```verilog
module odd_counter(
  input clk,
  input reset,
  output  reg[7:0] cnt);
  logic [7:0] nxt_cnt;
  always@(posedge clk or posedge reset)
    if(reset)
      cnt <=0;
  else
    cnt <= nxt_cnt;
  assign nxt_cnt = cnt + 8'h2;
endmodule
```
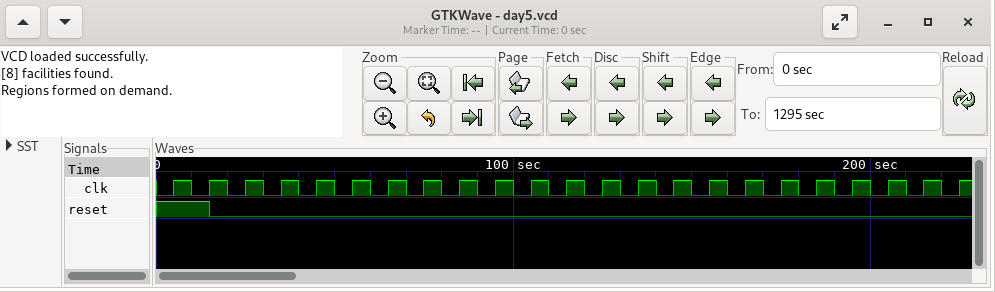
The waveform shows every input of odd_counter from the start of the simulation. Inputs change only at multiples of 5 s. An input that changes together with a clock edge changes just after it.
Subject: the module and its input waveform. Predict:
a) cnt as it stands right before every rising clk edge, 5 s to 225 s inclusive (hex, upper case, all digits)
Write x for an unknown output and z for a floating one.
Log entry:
00, 00, 00, 02, 04, 06, 08, 0A, 0C, 0E, 10, 12, 14, 16, 18, 1A, 1C, 1E, 20, 22, 24, 26, 28
